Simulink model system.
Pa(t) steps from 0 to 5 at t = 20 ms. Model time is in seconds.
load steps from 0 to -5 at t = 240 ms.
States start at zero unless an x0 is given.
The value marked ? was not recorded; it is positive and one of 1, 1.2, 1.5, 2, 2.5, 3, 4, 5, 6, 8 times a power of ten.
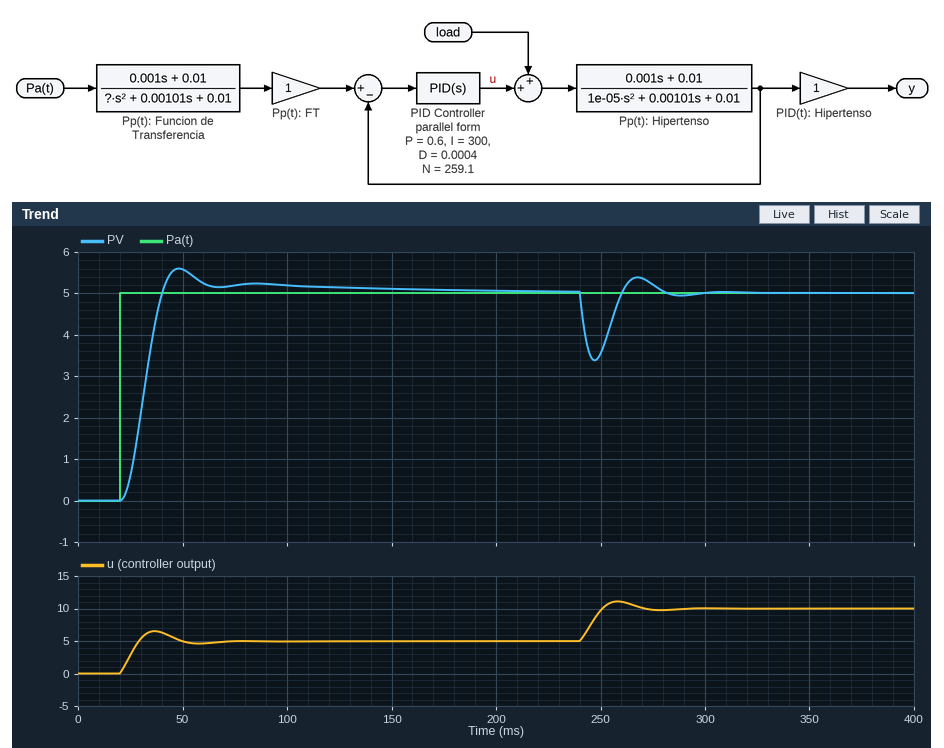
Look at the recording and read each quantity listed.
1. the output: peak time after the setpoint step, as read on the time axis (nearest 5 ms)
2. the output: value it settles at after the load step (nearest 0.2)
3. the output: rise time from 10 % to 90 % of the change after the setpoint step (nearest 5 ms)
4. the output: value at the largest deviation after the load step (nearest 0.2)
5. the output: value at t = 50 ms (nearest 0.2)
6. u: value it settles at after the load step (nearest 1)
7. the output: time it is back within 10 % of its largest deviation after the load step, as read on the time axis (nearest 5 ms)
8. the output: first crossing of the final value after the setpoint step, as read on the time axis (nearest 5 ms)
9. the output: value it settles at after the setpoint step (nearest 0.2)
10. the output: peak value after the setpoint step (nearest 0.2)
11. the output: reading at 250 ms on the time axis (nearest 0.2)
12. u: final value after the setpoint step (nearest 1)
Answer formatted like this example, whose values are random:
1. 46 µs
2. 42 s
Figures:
1. 50 ms
2. 5.0
3. 15 ms
4. 3.4
5. 5.6
6. 10
7. 275 ms
8. 40 ms
9. 5.0
10. 5.6
11. 3.6
12. 5
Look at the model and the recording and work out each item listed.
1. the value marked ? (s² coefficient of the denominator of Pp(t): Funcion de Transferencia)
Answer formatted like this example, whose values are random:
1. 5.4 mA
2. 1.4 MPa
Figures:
1. 8e-06
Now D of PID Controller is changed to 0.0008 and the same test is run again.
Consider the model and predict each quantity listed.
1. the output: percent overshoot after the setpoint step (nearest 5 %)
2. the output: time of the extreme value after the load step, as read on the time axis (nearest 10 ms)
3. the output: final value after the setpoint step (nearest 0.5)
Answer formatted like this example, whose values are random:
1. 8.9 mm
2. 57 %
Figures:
1. 10 %
2. 250 ms
3. 5.0
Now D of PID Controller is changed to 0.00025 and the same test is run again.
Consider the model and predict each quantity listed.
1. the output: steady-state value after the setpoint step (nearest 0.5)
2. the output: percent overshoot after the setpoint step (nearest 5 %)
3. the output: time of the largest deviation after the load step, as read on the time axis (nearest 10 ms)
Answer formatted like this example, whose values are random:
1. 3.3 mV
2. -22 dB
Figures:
1. 5.0
2. 10 %
3. 250 ms
